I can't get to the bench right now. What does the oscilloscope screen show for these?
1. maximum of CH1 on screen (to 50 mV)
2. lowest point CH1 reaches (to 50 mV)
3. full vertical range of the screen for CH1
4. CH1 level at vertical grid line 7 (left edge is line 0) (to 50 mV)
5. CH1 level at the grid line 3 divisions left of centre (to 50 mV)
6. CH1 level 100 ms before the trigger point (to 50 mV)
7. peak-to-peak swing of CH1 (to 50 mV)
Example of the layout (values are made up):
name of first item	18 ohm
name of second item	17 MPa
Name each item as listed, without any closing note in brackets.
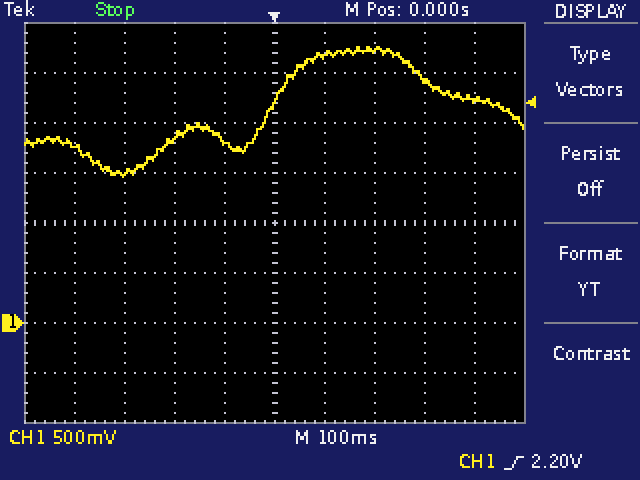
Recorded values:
maximum of CH1 on screen	2.75 V
lowest point CH1 reaches	1.45 V
full vertical range of the screen for CH1	4 V
CH1 level at vertical grid line 7 (left edge is line 0)	2.75 V
CH1 level at the grid line 3 divisions left of centre	1.50 V
CH1 level 100 ms before the trigger point	1.80 V
peak-to-peak swing of CH1	1.30 V
